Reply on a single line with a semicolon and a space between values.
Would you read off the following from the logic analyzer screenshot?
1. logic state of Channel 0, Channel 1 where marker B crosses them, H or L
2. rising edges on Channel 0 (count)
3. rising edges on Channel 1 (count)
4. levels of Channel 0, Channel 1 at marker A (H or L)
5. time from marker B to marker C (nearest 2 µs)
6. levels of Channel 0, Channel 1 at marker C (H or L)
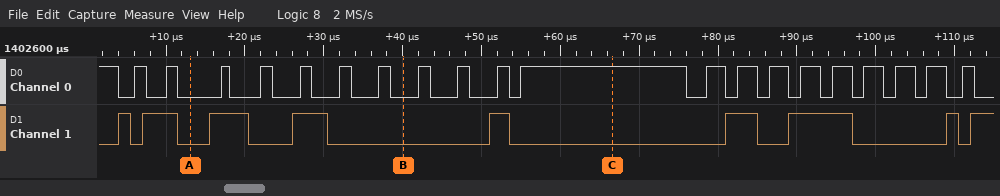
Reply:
Channel 0=L, Channel 1=L; 20; 9; Channel 0=L, Channel 1=L; 26 µs; Channel 0=H, Channel 1=L
